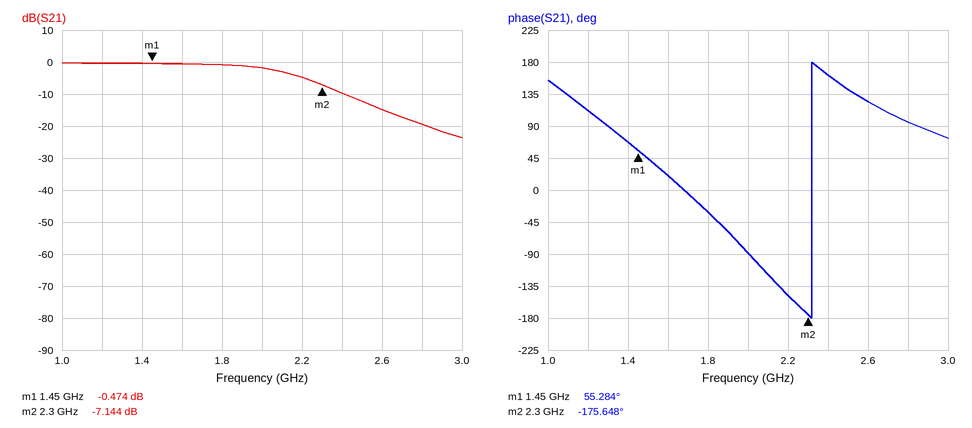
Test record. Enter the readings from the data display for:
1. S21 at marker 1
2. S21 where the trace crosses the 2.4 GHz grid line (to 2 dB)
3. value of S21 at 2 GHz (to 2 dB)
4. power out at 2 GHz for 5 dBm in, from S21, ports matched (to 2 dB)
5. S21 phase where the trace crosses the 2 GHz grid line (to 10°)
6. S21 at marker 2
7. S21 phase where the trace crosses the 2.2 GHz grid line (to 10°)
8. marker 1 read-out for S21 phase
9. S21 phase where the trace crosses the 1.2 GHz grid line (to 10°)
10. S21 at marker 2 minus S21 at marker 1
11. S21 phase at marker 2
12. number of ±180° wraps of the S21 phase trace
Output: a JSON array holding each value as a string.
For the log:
["-0.474 dB", "-10 dB", "-2 dB", "4 dBm", "-90°", "-7.144 dB", "-150°", "55.284°", "110°", "-6.670 dB", "-175.648°", "1"]
